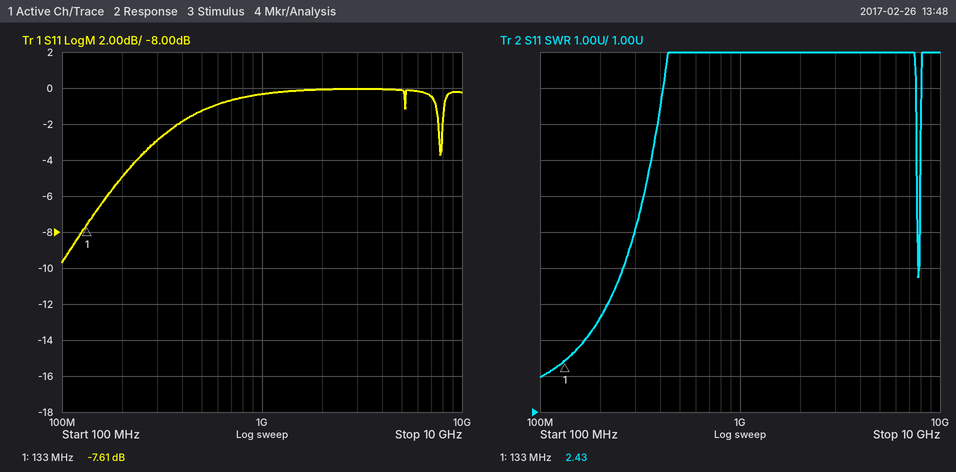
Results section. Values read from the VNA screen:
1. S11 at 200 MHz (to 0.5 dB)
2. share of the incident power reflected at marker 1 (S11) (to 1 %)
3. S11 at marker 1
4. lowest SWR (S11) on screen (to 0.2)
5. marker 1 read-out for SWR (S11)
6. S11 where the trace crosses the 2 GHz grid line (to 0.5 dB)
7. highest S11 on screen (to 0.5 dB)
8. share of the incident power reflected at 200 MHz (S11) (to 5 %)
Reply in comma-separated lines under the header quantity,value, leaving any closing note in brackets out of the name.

quantity,value
S11 at 200 MHz,-5.0 dB
share of the incident power reflected at marker 1 (S11),17 %
S11 at marker 1,-7.61 dB
lowest SWR (S11) on screen,2.0
marker 1 read-out for SWR,2.43
S11 where the trace crosses the 2 GHz grid line,0.0 dB
highest S11 on screen,0.0 dB
share of the incident power reflected at 200 MHz (S11),30 %
